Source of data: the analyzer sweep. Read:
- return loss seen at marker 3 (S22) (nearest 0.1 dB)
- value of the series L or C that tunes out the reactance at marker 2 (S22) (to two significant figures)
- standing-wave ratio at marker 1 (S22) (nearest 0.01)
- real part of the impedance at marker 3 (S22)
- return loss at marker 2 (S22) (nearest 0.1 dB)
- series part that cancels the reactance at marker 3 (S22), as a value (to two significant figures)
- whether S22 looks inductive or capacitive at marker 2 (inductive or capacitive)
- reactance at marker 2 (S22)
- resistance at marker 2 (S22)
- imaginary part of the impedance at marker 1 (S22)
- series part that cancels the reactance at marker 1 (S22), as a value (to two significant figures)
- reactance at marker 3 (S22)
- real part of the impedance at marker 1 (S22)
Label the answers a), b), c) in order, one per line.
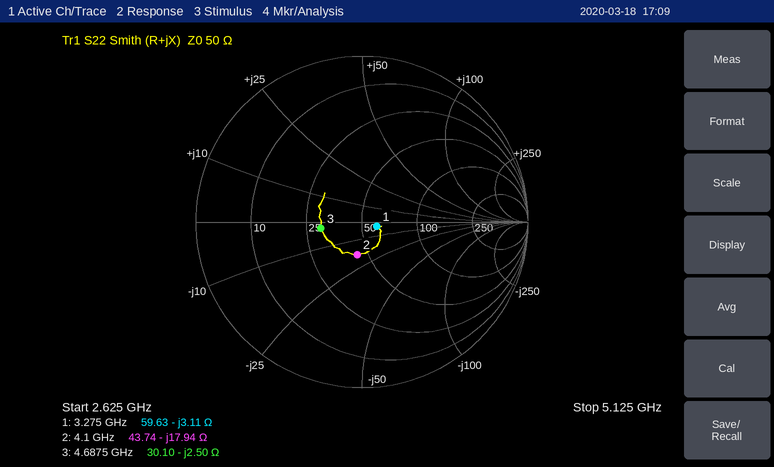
a) 12.0 dB
b) 700 pH
c) 1.20
d) 30.10 Ω
e) 14.0 dB
f) 85 pH
g) capacitive
h) -17.94 Ω
i) 43.74 Ω
j) -3.11 Ω
k) 150 pH
l) -2.50 Ω
m) 59.63 Ω
